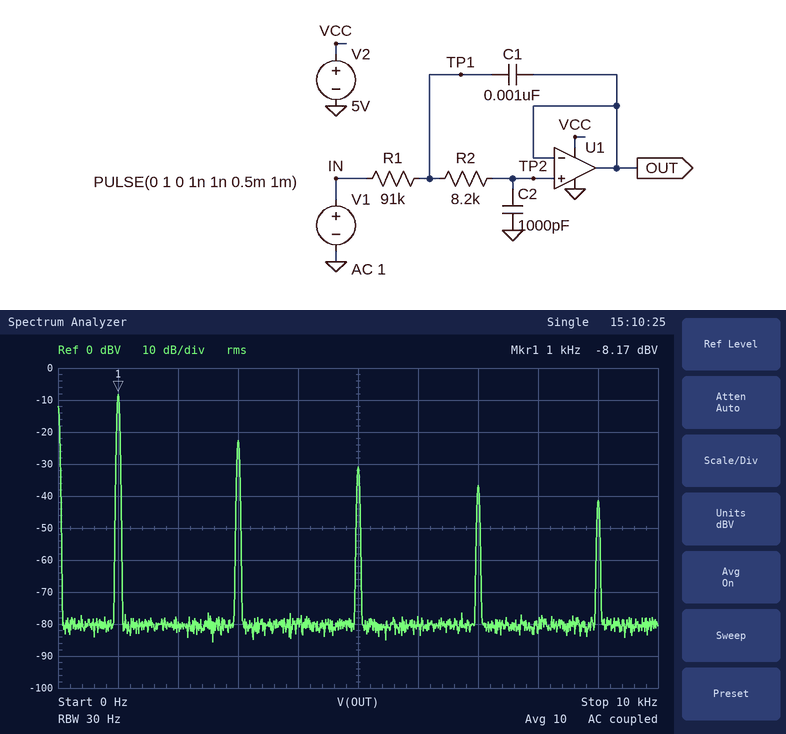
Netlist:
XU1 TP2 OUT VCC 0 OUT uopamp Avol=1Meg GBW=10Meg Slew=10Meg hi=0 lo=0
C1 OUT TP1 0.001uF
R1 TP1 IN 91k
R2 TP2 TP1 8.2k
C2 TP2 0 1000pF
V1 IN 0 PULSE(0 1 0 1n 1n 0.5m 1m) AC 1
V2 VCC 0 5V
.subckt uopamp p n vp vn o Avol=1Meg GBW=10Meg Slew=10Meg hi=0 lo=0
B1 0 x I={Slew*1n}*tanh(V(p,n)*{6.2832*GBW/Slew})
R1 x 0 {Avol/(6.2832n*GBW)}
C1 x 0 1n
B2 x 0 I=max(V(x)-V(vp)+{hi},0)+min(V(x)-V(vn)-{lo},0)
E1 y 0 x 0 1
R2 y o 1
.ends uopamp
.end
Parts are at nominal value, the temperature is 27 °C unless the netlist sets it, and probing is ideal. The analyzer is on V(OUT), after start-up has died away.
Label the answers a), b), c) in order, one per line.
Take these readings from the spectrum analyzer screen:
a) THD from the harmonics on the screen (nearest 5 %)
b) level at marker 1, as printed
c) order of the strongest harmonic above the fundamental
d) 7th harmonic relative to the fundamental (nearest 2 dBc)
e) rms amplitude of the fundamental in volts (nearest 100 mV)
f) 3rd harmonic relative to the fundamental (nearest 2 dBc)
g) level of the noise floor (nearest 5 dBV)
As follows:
a) 20 %
b) -8.17 dBV
c) 3
d) -28 dBc
e) 400 mV
f) -14 dBc
g) -80 dBV
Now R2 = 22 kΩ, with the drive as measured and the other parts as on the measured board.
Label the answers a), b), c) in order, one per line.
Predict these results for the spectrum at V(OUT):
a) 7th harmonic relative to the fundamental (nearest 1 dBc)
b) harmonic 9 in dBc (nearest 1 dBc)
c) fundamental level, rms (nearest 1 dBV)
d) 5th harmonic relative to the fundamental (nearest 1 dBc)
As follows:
a) -31 dBc
b) -36 dBc
c) -8 dBV
d) -24 dBc
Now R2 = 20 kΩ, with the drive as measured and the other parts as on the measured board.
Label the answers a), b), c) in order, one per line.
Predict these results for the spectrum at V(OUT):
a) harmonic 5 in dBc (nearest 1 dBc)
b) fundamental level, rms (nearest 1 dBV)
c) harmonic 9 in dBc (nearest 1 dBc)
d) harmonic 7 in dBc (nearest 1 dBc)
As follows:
a) -24 dBc
b) -8 dBV
c) -36 dBc
d) -30 dBc
